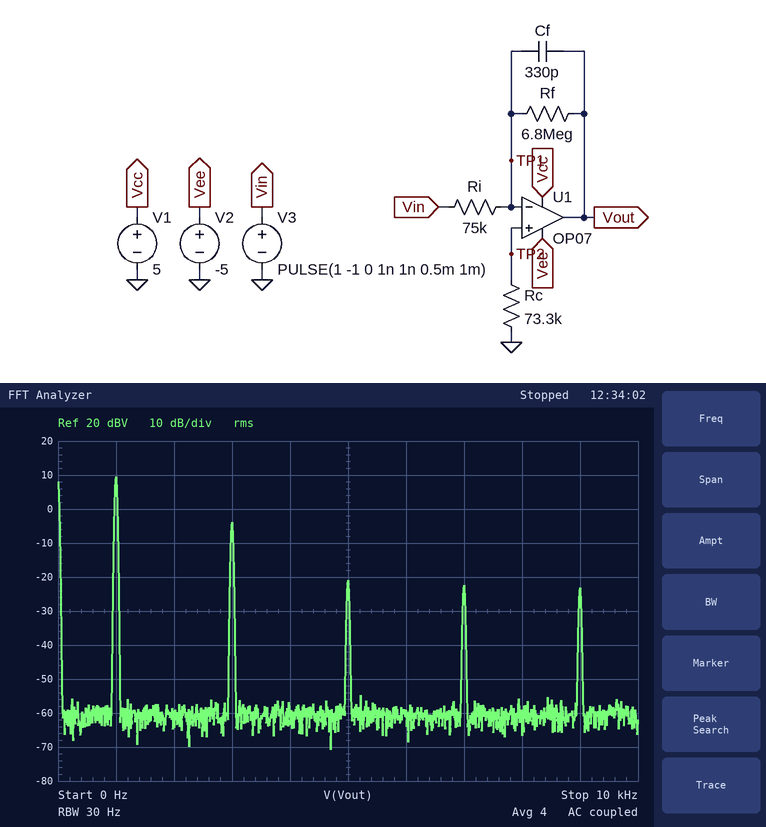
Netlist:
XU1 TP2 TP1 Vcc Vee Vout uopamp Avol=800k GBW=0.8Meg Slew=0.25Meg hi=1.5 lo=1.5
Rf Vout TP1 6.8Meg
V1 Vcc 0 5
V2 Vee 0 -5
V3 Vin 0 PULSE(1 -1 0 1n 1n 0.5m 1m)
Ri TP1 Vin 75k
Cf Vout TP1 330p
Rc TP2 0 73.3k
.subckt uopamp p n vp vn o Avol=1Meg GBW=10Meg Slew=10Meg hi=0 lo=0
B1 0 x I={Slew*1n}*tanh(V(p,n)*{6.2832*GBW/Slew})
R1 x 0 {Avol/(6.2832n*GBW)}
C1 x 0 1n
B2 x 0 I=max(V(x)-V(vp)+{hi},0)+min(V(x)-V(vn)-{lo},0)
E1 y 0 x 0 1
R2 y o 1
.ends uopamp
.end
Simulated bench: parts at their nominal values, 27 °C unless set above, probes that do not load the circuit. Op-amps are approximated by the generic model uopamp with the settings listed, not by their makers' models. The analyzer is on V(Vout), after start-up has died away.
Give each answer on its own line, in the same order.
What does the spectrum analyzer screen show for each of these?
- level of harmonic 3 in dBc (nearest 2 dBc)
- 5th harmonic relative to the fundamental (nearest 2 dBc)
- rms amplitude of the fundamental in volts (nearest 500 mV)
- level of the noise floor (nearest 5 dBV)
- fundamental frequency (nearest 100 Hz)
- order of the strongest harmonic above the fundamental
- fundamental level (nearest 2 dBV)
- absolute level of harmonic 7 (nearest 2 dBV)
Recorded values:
-14 dBc
-30 dBc
3.0 V
-60 dBV
1.0 kHz
3
10 dBV
-22 dBV
